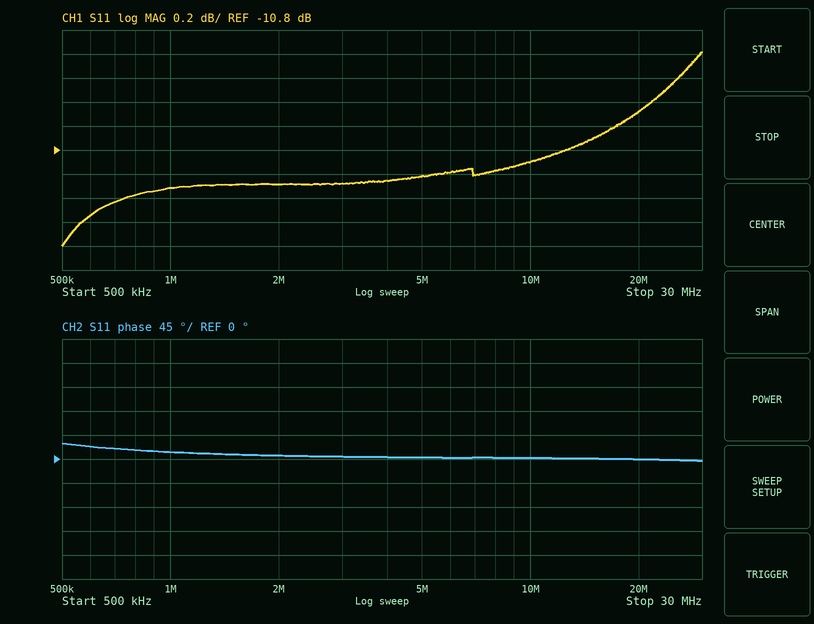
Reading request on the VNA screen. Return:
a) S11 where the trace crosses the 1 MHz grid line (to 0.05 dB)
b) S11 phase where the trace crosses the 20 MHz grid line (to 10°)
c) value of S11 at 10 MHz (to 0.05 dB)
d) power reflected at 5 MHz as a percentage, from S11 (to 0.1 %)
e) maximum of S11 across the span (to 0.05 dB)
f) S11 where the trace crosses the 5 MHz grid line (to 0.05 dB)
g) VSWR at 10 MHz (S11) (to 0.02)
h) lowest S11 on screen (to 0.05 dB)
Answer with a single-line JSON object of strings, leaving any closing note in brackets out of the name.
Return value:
{"S11 where the trace crosses the 1 MHz grid line": "-11.10 dB", "S11 phase where the trace crosses the 20 MHz grid line": "0°", "value of S11 at 10 MHz": "-10.90 dB", "power reflected at 5 MHz as a percentage, from S11": "7.9 %", "maximum of S11 across the span": "-10.00 dB", "S11 where the trace crosses the 5 MHz grid line": "-11.00 dB", "VSWR at 10 MHz (S11)": "1.80", "lowest S11 on screen": "-11.60 dB"}
